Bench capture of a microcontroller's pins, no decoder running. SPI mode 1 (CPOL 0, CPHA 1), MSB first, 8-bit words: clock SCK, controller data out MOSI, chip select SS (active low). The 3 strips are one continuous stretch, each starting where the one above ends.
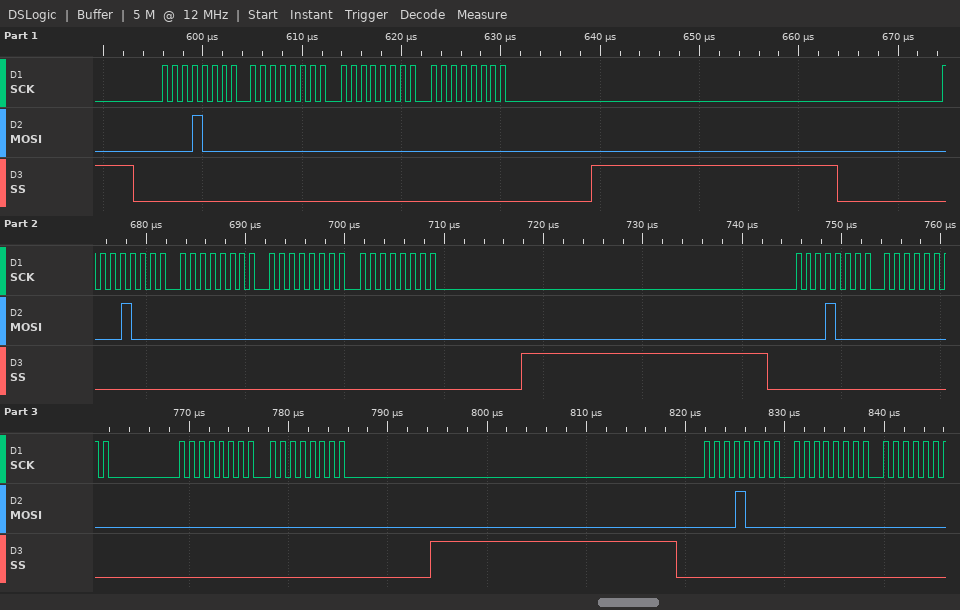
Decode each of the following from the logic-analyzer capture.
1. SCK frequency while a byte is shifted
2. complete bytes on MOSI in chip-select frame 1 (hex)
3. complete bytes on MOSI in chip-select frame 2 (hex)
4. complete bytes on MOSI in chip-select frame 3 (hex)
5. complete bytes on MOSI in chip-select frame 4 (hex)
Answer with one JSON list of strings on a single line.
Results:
["1 MHz", "10 00 00 00", "10 00 00 00", "10 00 00 00", "10 00"]
